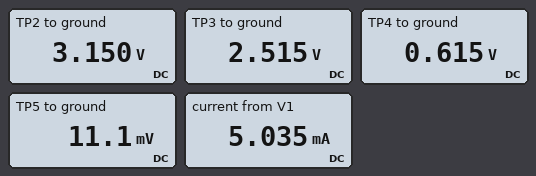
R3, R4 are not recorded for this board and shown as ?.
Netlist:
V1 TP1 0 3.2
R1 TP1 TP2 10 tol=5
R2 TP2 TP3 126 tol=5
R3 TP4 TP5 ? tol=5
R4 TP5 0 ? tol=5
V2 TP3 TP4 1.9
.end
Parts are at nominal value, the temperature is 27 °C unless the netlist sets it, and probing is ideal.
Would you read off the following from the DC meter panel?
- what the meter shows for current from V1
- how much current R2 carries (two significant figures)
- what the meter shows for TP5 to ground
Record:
5.035 mA
5.0 mA
11.1 mV
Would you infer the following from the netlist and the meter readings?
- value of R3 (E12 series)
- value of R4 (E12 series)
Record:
120 Ω
2.2 Ω
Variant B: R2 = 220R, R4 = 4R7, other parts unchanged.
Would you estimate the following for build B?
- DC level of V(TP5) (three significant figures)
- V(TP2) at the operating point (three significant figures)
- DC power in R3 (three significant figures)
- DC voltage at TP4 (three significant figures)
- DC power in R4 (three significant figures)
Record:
17.2 mV
3.16 V
1.61 mW
457 mV
63.1 µW
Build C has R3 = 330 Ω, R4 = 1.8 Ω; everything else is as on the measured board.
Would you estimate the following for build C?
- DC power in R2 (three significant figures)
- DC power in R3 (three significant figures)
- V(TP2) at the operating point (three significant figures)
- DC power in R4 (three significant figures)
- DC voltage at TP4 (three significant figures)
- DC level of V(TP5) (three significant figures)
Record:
973 µW
2.55 mW
3.17 V
13.9 µW
922 mV
5.00 mV
